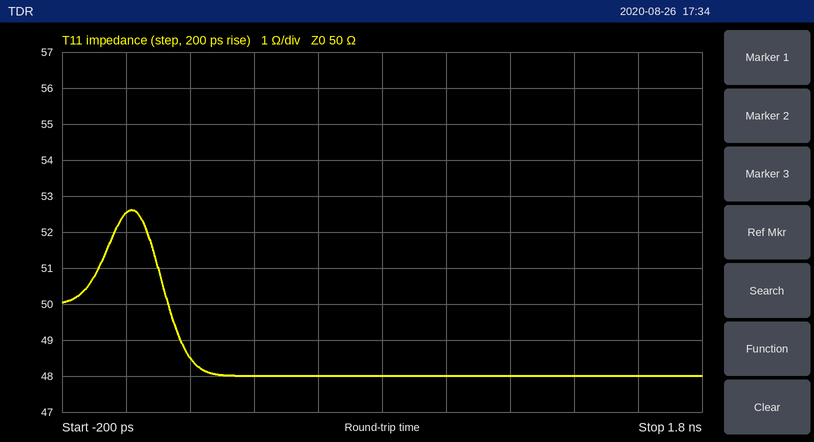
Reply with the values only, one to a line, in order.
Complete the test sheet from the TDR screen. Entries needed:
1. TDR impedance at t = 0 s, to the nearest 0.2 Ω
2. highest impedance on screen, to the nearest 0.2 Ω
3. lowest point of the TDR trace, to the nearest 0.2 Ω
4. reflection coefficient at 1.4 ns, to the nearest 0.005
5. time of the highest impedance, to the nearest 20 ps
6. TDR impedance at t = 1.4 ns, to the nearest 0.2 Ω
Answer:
52.6 Ω
52.6 Ω
48.0 Ω
-0.020
20 ps
48.0 Ω
